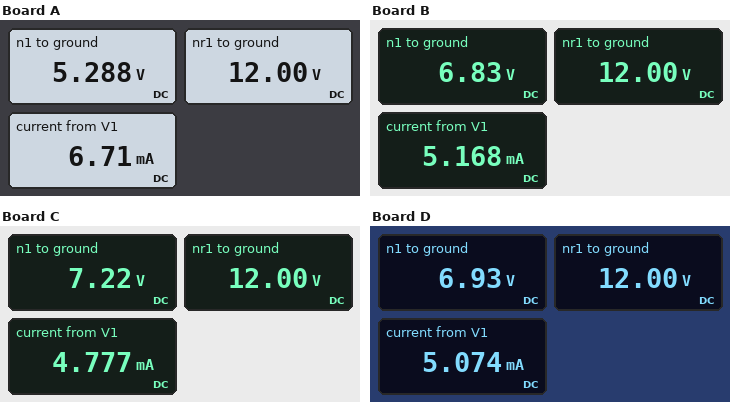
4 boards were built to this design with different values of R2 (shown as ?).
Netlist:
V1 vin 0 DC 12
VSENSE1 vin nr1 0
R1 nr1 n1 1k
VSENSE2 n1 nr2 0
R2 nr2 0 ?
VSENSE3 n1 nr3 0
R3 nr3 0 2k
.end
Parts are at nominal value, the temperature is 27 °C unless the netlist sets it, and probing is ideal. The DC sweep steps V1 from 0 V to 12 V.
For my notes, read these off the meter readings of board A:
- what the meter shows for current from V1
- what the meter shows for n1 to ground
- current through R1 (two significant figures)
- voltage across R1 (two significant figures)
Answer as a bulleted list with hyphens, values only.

- 6.71 mA
- 5.288 V
- 6.7 mA
- 6.7 V
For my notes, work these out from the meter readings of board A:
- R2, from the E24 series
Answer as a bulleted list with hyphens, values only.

- 1.3 kΩ
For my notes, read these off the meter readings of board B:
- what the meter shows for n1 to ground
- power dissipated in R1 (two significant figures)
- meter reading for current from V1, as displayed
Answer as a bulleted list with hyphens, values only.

- 6.83 V
- 27 mW
- 5.168 mA
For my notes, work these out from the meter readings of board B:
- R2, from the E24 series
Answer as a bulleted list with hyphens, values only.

- 3.9 kΩ
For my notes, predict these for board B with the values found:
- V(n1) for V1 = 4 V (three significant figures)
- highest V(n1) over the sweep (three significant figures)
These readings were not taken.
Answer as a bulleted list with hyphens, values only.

- 2.28 V
- 6.83 V
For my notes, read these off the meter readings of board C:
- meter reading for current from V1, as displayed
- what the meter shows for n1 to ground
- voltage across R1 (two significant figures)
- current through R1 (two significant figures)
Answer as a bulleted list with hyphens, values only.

- 4.777 mA
- 7.22 V
- 4.8 V
- 4.8 mA
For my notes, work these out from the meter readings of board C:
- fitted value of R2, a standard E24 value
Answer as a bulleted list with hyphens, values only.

- 6.2 kΩ
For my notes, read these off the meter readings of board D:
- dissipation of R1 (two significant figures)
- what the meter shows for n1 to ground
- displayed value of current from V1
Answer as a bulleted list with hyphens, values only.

- 26 mW
- 6.93 V
- 5.074 mA
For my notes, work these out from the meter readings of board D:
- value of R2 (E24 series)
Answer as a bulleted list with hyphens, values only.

- 4.3 kΩ
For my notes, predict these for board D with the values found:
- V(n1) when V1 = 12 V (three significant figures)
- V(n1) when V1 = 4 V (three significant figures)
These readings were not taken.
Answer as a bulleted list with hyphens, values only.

- 6.93 V
- 2.31 V
